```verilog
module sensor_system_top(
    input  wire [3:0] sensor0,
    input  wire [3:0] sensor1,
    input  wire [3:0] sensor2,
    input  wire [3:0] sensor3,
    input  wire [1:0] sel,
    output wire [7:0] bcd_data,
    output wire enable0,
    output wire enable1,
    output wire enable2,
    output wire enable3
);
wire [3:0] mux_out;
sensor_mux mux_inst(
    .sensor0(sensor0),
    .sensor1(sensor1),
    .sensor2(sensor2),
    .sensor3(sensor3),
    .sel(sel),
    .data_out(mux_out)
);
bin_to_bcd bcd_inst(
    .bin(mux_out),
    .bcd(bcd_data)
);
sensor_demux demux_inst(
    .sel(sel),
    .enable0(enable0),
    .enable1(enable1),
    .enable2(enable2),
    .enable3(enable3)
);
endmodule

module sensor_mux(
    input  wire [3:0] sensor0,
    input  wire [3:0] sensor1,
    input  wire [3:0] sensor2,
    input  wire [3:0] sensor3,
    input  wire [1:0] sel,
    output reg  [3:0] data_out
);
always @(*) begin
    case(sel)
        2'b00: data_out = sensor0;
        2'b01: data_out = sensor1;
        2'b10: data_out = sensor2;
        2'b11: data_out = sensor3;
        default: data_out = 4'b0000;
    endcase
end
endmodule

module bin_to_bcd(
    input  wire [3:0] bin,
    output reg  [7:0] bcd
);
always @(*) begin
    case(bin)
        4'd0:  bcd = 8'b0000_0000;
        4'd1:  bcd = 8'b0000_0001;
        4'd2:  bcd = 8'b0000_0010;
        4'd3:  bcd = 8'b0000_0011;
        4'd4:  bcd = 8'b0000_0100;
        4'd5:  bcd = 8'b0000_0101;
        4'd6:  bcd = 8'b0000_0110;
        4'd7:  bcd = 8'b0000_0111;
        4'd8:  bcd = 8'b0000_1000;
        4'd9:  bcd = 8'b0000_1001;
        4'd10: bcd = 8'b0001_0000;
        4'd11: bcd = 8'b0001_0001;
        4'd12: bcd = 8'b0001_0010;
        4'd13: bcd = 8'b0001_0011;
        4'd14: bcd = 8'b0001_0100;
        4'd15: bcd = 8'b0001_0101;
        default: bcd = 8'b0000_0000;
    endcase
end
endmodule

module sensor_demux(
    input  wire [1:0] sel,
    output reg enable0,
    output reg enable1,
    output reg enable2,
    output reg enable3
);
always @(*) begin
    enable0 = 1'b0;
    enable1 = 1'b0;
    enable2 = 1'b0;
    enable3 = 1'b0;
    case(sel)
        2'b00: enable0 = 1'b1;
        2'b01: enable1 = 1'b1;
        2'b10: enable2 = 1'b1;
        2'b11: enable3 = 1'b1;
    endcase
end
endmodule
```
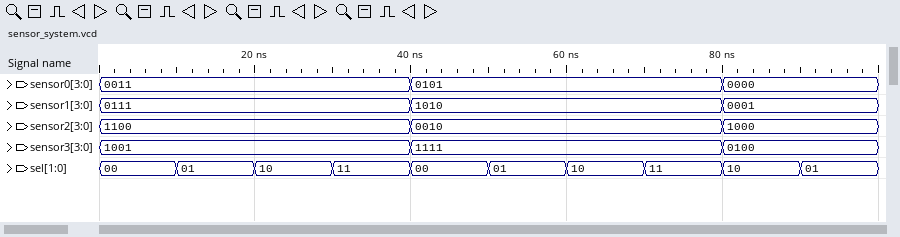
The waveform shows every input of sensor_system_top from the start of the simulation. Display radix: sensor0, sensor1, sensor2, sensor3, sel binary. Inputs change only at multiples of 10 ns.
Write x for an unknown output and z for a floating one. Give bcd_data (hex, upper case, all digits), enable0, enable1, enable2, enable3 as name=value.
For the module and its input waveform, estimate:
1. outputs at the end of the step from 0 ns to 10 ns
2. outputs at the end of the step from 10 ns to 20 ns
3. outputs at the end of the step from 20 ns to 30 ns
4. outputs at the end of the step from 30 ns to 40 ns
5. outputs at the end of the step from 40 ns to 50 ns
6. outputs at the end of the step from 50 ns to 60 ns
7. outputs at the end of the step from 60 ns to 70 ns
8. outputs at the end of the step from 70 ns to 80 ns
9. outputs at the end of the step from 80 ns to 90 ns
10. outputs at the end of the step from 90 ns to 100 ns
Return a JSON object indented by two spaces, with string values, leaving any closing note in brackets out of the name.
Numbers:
{
  "outputs at the end of the step from 0 ns to 10 ns": "bcd_data=03, enable0=1, enable1=0, enable2=0, enable3=0",
  "outputs at the end of the step from 10 ns to 20 ns": "bcd_data=07, enable0=0, enable1=1, enable2=0, enable3=0",
  "outputs at the end of the step from 20 ns to 30 ns": "bcd_data=12, enable0=0, enable1=0, enable2=1, enable3=0",
  "outputs at the end of the step from 30 ns to 40 ns": "bcd_data=09, enable0=0, enable1=0, enable2=0, enable3=1",
  "outputs at the end of the step from 40 ns to 50 ns": "bcd_data=05, enable0=1, enable1=0, enable2=0, enable3=0",
  "outputs at the end of the step from 50 ns to 60 ns": "bcd_data=10, enable0=0, enable1=1, enable2=0, enable3=0",
  "outputs at the end of the step from 60 ns to 70 ns": "bcd_data=02, enable0=0, enable1=0, enable2=1, enable3=0",
  "outputs at the end of the step from 70 ns to 80 ns": "bcd_data=15, enable0=0, enable1=0, enable2=0, enable3=1",
  "outputs at the end of the step from 80 ns to 90 ns": "bcd_data=08, enable0=0, enable1=0, enable2=1, enable3=0",
  "outputs at the end of the step from 90 ns to 100 ns": "bcd_data=01, enable0=0, enable1=1, enable2=0, enable3=0"
}
